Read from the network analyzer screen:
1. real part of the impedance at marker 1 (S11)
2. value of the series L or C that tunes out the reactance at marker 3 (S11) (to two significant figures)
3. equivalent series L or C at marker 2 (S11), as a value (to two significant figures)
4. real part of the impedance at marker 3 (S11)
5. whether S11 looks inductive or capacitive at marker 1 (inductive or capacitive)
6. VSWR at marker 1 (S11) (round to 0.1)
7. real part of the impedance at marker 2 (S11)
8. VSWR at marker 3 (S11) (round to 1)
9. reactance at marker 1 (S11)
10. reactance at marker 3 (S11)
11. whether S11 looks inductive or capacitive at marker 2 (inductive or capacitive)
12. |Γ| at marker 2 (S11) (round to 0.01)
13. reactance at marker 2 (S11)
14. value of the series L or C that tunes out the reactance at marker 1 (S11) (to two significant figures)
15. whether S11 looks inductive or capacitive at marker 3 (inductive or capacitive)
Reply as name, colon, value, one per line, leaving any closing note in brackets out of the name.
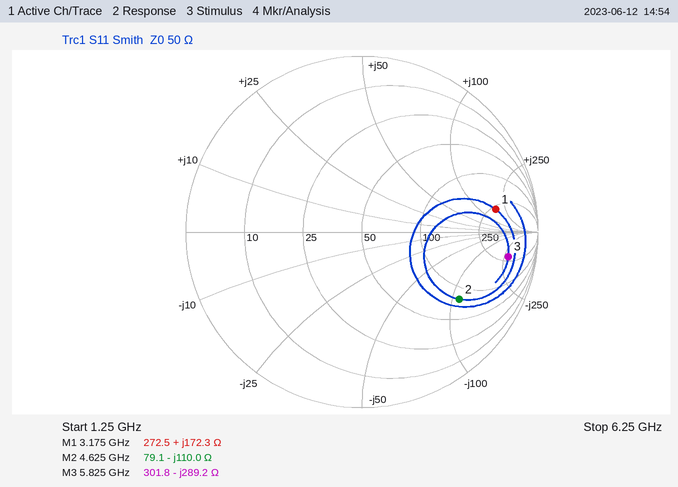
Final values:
real part of the impedance at marker 1: 272.5 Ω
value of the series L or C that tunes out the reactance at marker 3 (S11): 7.9 nH
equivalent series L or C at marker 2 (S11), as a value: 310 fF
real part of the impedance at marker 3: 301.8 Ω
whether S11 looks inductive or capacitive at marker 1: inductive
VSWR at marker 1 (S11): 7.7
real part of the impedance at marker 2: 79.1 Ω
VSWR at marker 3 (S11): 12
reactance at marker 1: +172.3 Ω
reactance at marker 3: -289.2 Ω
whether S11 looks inductive or capacitive at marker 2: capacitive
|Γ| at marker 2 (S11): 0.67
reactance at marker 2: -110.0 Ω
value of the series L or C that tunes out the reactance at marker 1 (S11): 290 fF
whether S11 looks inductive or capacitive at marker 3: capacitive
